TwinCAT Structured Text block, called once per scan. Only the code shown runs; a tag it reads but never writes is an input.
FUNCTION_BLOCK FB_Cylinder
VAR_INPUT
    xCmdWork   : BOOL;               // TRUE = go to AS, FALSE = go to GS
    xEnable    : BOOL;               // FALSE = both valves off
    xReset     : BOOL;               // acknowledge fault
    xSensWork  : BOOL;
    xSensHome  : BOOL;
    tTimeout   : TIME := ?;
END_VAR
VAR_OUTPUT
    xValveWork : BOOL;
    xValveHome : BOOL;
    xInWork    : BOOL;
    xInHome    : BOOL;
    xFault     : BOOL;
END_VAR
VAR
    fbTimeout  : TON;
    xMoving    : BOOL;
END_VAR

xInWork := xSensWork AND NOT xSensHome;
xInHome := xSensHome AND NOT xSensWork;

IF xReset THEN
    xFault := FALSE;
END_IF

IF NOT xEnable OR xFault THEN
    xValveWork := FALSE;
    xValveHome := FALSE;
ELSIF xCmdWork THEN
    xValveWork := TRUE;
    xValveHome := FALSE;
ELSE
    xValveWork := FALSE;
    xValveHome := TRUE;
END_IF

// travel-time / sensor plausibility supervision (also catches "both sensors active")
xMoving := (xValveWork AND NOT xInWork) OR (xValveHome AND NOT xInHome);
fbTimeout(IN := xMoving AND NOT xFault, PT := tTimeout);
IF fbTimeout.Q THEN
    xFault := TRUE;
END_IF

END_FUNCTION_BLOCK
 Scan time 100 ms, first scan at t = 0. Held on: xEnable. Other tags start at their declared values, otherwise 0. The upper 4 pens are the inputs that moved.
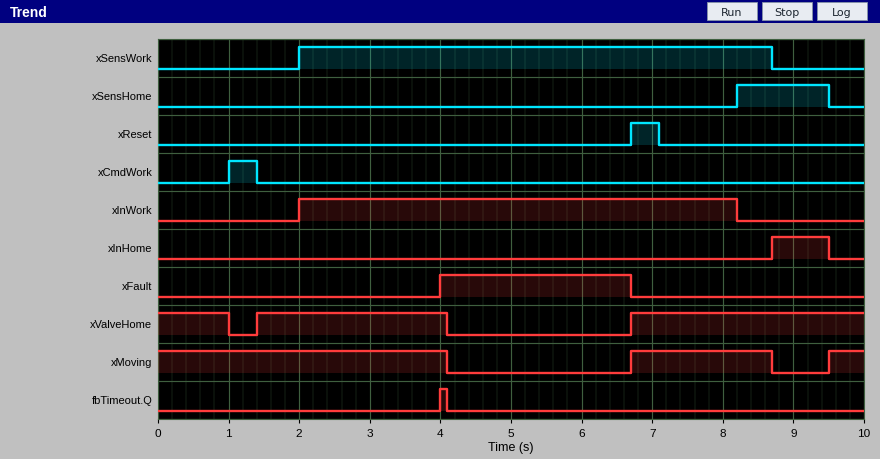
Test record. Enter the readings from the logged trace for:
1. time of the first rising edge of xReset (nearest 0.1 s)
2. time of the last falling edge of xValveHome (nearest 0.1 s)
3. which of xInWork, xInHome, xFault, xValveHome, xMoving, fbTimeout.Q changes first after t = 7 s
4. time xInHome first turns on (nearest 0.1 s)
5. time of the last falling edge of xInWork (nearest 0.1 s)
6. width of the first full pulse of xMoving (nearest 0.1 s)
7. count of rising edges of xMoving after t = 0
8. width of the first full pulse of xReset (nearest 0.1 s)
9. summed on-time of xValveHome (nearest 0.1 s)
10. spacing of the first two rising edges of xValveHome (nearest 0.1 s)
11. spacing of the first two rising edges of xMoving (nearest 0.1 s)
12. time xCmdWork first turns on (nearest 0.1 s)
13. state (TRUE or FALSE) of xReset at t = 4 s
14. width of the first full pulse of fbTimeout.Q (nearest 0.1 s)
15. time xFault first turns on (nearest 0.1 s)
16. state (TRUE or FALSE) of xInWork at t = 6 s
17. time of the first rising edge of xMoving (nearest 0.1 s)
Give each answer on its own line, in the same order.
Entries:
6.7 s
4.1 s
xInWork
8.7 s
8.2 s
2.0 s
2
0.4 s
7.0 s
5.3 s
2.8 s
1.0 s
FALSE
0.1 s
4.0 s
TRUE
6.7 s
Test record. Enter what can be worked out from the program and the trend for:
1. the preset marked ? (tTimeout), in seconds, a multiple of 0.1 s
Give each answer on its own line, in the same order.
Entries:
4.0 s
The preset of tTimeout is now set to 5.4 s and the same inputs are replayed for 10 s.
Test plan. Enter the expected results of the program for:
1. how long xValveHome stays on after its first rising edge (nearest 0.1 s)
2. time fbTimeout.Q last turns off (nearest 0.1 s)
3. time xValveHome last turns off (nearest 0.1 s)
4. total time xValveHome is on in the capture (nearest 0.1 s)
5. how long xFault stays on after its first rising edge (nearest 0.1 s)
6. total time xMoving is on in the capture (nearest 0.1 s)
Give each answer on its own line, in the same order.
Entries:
4.1 s
5.5 s
5.5 s
8.4 s
1.3 s
8.0 s
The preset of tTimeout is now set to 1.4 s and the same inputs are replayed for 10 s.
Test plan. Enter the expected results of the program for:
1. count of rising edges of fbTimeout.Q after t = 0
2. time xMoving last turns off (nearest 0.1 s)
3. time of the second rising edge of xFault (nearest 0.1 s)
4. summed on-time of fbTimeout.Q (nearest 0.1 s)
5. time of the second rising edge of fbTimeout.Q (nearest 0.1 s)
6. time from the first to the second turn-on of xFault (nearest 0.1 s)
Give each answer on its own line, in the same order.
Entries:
2
8.2 s
8.1 s
0.2 s
8.1 s
6.7 s
